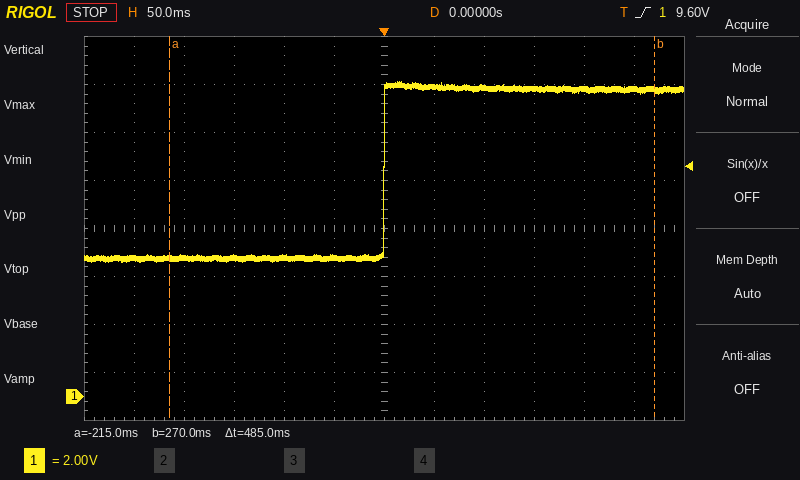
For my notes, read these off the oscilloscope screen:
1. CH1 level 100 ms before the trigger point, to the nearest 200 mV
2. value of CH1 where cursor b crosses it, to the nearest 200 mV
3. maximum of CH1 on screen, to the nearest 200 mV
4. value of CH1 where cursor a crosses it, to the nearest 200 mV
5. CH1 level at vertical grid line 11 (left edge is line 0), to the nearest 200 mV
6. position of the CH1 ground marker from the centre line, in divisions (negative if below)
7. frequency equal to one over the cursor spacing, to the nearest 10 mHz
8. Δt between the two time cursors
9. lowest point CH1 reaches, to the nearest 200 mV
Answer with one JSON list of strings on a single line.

["5.8 V", "12.8 V", "13.2 V", "5.8 V", "12.8 V", "-3.5 div", "2.06 Hz", "485 ms", "5.6 V"]
